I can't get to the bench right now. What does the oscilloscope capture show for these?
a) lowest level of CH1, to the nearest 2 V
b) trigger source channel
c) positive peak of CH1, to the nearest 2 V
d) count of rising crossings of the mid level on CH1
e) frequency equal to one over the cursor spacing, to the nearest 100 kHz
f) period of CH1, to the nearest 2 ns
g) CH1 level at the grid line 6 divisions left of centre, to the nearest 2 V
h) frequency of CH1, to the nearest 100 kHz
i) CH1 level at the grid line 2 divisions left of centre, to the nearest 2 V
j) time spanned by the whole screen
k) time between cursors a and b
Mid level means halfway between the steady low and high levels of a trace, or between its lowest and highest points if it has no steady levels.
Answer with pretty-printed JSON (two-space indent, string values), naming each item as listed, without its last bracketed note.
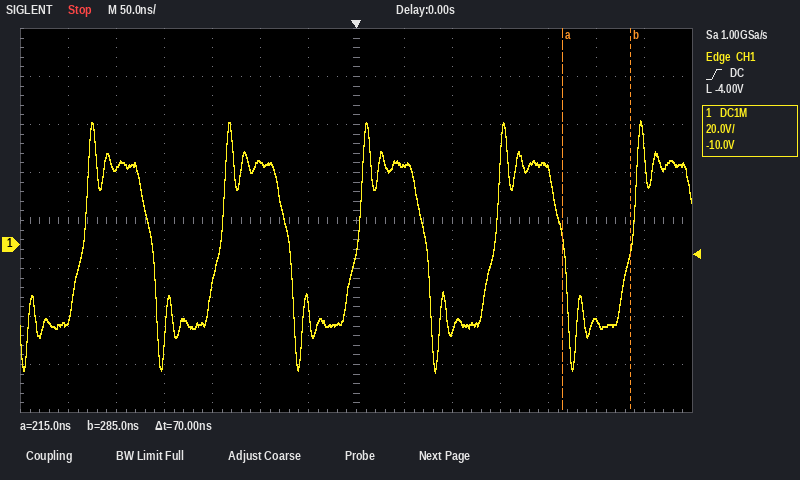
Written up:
{
  "lowest level of CH1, to the nearest 2 V": "-54 V",
  "trigger source channel": "CH1",
  "positive peak of CH1, to the nearest 2 V": "52 V",
  "count of rising crossings of the mid level on CH1": "5",
  "frequency equal to one over the cursor spacing, to the nearest 100 kHz": "14.3 MHz",
  "period of CH1, to the nearest 2 ns": "142 ns",
  "CH1 level at the grid line 6 divisions left of centre, to the nearest 2 V": "-32 V",
  "frequency of CH1, to the nearest 100 kHz": "7.0 MHz",
  "CH1 level at the grid line 2 divisions left of centre, to the nearest 2 V": "34 V",
  "time spanned by the whole screen": "700 ns",
  "time between cursors a and b": "70 ns"
}
